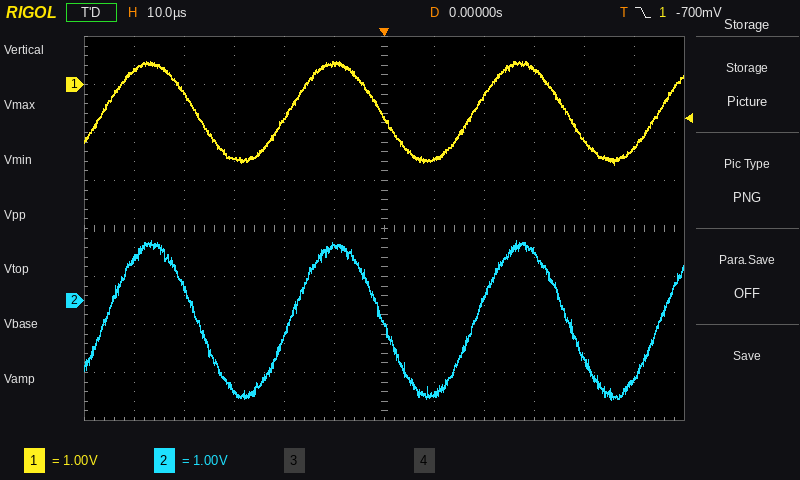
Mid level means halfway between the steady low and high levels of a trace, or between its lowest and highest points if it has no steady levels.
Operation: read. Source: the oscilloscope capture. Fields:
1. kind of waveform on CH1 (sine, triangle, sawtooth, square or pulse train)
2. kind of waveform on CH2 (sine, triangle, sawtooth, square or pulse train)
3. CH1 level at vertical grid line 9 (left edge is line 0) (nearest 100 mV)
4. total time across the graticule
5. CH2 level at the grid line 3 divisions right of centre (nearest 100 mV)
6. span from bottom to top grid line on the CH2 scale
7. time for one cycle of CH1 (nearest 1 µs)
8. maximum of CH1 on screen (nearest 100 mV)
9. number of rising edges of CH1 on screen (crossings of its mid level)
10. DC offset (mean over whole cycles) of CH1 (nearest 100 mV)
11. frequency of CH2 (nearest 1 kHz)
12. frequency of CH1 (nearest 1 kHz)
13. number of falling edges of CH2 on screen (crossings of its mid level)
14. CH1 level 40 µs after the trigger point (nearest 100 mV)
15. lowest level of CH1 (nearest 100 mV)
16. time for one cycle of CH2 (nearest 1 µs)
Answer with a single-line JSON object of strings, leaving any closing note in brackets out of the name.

{"kind of waveform on CH1": "sine", "kind of waveform on CH2": "sine", "CH1 level at vertical grid line 9 (left edge is line 0)": "300 mV", "total time across the graticule": "120 µs", "CH2 level at the grid line 3 divisions right of centre": "1.0 V", "span from bottom to top grid line on the CH2 scale": "8 V", "time for one cycle of CH1": "37 µs", "maximum of CH1 on screen": "500 mV", "number of rising edges of CH1 on screen": "4", "DC offset (mean over whole cycles) of CH1": "-600 mV", "frequency of CH2": "27 kHz", "frequency of CH1": "27 kHz", "number of falling edges of CH2 on screen": "3", "CH1 level 40 µs after the trigger point": "-1.2 V", "lowest level of CH1": "-1.7 V", "time for one cycle of CH2": "37 µs"}
